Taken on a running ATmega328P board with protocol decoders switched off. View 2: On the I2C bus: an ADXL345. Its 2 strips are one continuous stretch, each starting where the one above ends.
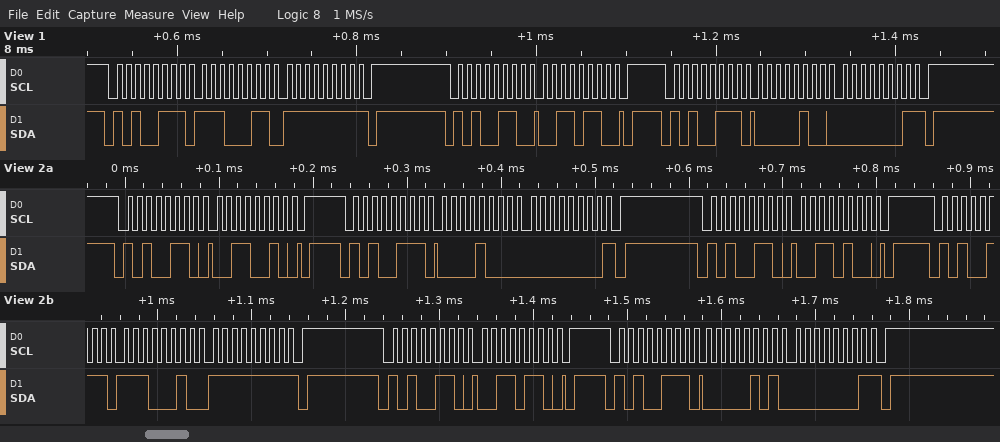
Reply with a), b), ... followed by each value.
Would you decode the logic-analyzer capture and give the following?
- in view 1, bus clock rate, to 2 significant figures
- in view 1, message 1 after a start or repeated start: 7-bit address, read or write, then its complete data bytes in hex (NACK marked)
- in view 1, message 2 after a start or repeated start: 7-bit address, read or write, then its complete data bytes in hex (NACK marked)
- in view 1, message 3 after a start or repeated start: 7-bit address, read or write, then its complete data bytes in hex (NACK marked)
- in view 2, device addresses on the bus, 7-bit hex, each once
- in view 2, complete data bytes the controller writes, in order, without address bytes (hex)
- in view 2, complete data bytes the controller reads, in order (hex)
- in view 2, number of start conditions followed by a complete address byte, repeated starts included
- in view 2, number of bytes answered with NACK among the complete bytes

a) 100 kHz
b) 0x53 read: E3 FF NACK
c) 0x53 write: 36
d) 0x53 read: 04 01 NACK
e) 0x53
f) 32 34 36
g) 08 00 E2 FF 05 01
h) 6
i) 3
